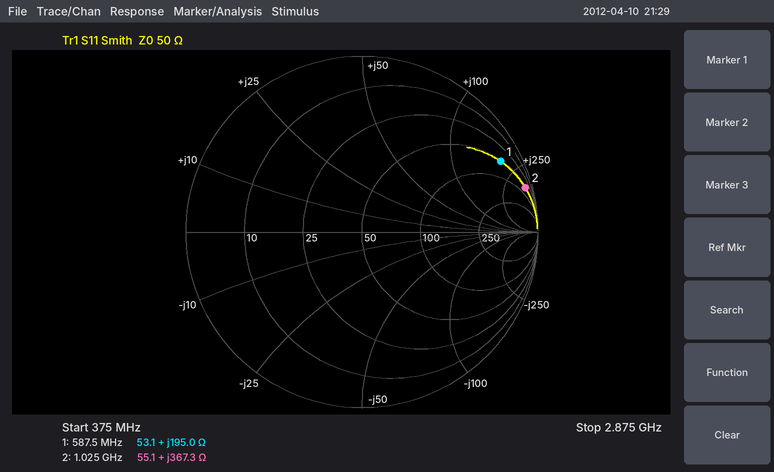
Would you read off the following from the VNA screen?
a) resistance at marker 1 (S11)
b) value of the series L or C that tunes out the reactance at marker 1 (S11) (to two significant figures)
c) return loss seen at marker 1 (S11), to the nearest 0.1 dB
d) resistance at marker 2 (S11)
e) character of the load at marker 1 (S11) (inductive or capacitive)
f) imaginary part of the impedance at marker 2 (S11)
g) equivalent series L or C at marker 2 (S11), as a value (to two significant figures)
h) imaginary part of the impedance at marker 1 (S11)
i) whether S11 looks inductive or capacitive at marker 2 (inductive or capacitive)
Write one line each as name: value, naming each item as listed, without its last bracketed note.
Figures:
resistance at marker 1: 53.1 Ω
value of the series L or C that tunes out the reactance at marker 1 (S11): 1.4 pF
return loss seen at marker 1 (S11), to the nearest 0.1 dB: 1.1 dB
resistance at marker 2: 55.1 Ω
character of the load at marker 1 (S11): inductive
imaginary part of the impedance at marker 2: +367.3 Ω
equivalent series L or C at marker 2 (S11), as a value: 57 nH
imaginary part of the impedance at marker 1: +195.0 Ω
whether S11 looks inductive or capacitive at marker 2: inductive
